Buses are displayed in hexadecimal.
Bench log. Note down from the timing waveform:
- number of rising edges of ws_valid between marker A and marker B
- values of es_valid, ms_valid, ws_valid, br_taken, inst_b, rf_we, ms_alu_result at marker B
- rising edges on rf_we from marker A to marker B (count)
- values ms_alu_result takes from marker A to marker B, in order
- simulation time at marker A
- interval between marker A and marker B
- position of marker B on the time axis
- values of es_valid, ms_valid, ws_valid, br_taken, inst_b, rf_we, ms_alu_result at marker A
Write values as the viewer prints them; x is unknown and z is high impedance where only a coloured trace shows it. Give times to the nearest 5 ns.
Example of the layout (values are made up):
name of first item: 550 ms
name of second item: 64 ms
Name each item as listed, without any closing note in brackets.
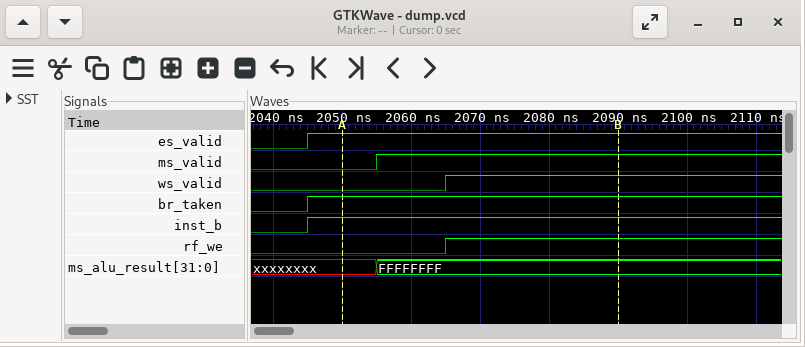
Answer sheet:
number of rising edges of ws_valid between marker A and marker B: 1
values of es_valid, ms_valid, ws_valid, br_taken, inst_b, rf_we, ms_alu_result at marker B: es_valid=1, ms_valid=1, ws_valid=1, br_taken=1, inst_b=1, rf_we=1, ms_alu_result=FFFFFFFF
rising edges on rf_we from marker A to marker B: 1
values ms_alu_result takes from marker A to marker B, in order: xxxxxxxx, FFFFFFFF
simulation time at marker A: 2050 ns
interval between marker A and marker B: 40 ns
position of marker B on the time axis: 2090 ns
values of es_valid, ms_valid, ws_valid, br_taken, inst_b, rf_we, ms_alu_result at marker A: es_valid=1, ms_valid=0, ws_valid=0, br_taken=1, inst_b=1, rf_we=0, ms_alu_result=xxxxxxxx
